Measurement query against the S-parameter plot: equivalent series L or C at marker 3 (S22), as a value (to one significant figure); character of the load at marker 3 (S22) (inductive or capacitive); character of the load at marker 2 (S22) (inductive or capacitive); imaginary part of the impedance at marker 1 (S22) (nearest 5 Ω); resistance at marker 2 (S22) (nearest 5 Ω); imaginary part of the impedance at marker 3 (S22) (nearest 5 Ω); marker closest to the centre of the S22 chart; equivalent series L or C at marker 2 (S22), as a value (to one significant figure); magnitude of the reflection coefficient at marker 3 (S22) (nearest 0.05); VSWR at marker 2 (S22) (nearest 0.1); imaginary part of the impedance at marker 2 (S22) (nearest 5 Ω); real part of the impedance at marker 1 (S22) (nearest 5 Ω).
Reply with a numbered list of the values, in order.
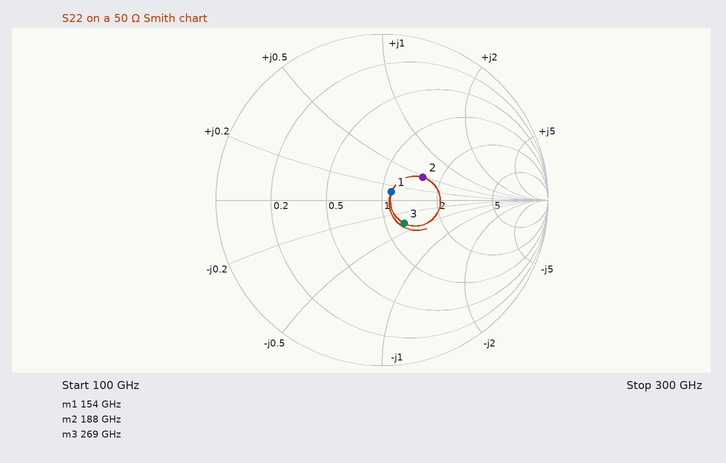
1. 30 fF
2. capacitive
3. inductive
4. +5 Ω
5. 80 Ω
6. -20 Ω
7. marker 1
8. 20 pH
9. 0.20
10. 1.8
11. +25 Ω
12. 55 Ω
